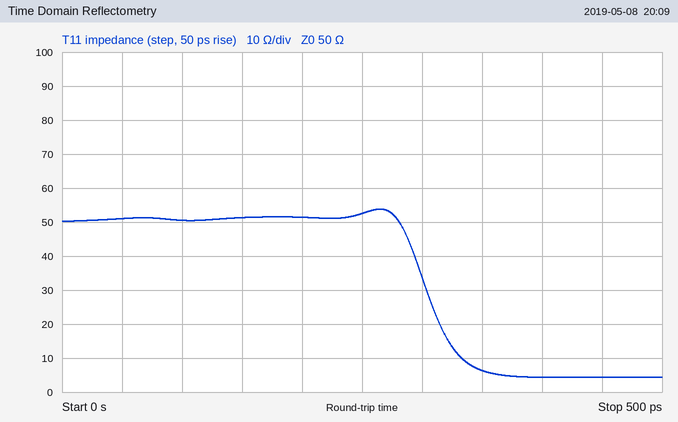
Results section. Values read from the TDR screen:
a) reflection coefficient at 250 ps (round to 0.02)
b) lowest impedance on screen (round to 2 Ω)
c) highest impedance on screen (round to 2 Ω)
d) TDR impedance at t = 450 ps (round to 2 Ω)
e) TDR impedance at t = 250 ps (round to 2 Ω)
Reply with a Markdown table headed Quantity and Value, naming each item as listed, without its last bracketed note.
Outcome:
| Quantity | Value |
|---|---|
| reflection coefficient at 250 ps | +0.02 |
| lowest impedance on screen | 4 Ω |
| highest impedance on screen | 54 Ω |
| TDR impedance at t = 450 ps | 4 Ω |
| TDR impedance at t = 250 ps | 52 Ω |
